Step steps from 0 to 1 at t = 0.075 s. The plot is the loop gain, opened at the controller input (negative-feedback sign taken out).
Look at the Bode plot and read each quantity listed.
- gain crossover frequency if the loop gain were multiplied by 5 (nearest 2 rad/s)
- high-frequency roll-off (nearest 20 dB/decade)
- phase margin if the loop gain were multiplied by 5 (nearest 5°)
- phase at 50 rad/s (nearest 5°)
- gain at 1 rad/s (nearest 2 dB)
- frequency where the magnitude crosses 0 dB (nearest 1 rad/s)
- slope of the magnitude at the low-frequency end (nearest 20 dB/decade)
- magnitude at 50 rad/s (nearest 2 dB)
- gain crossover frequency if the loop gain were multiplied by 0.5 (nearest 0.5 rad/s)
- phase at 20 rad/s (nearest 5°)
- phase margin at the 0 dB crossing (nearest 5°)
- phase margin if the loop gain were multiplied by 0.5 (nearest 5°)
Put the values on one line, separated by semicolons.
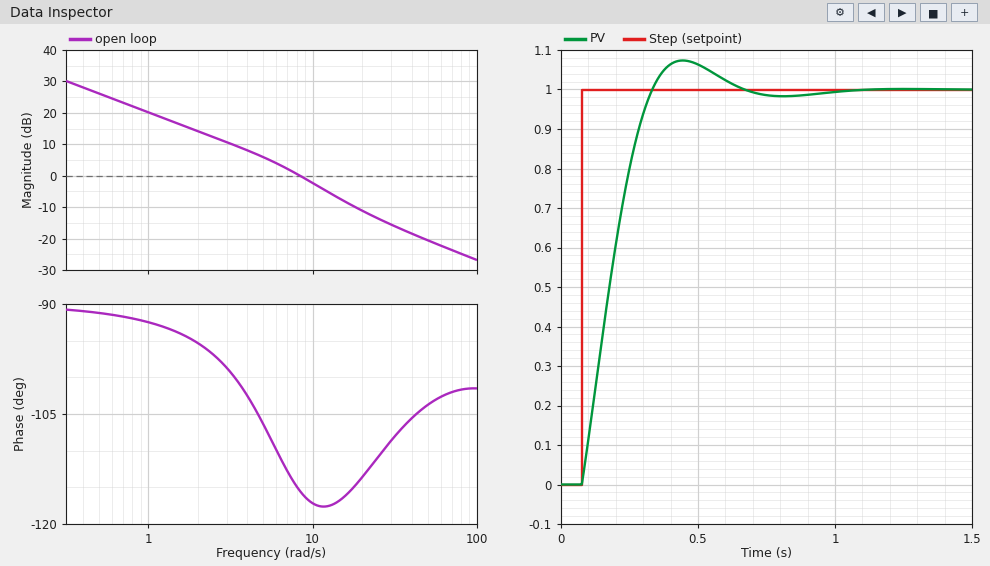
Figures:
26 rad/s; -20 dB/decade; 70°; -105°; 20 dB; 8 rad/s; -20 dB/decade; -20 dB; 5.0 rad/s; -115°; 65°; 75°
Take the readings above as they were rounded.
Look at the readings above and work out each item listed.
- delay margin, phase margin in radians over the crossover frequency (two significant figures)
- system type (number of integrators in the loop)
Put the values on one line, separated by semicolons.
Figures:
0.14 s; 1
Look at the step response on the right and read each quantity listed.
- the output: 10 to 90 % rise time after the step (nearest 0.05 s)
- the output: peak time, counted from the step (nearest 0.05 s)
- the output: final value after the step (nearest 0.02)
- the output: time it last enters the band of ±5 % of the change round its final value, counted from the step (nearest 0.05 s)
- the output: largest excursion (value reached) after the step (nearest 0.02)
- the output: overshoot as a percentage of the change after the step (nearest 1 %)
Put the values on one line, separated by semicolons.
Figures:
0.20 s; 0.35 s; 1.00; 0.45 s; 1.08; 7 %
